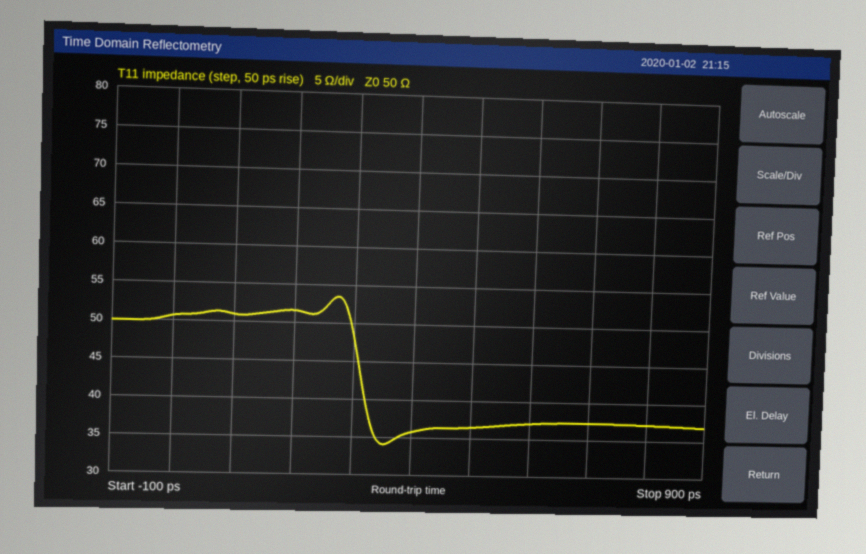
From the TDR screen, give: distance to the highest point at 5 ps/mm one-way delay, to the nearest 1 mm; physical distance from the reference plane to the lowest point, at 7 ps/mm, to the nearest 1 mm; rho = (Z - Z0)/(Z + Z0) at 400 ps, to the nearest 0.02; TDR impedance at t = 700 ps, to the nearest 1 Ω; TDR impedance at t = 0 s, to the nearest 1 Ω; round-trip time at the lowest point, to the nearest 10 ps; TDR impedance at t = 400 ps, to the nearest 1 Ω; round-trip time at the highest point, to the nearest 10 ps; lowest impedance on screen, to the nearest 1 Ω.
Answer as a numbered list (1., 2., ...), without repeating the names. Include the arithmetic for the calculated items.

1. 270 ps / 2 / 5 ps/mm ≈ 27 mm
2. 350 ps / 2 / 7 ps/mm ≈ 25 mm
3. (36 − 50)/(36 + 50) ≈ -0.16
4. 37 Ω
5. 51 Ω
6. 350 ps
7. 36 Ω
8. 270 ps
9. 34 Ω
